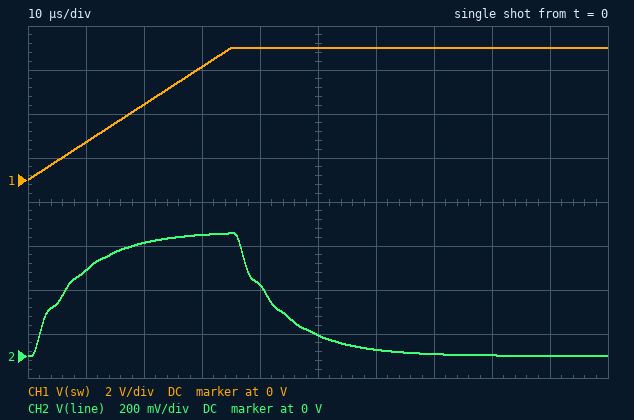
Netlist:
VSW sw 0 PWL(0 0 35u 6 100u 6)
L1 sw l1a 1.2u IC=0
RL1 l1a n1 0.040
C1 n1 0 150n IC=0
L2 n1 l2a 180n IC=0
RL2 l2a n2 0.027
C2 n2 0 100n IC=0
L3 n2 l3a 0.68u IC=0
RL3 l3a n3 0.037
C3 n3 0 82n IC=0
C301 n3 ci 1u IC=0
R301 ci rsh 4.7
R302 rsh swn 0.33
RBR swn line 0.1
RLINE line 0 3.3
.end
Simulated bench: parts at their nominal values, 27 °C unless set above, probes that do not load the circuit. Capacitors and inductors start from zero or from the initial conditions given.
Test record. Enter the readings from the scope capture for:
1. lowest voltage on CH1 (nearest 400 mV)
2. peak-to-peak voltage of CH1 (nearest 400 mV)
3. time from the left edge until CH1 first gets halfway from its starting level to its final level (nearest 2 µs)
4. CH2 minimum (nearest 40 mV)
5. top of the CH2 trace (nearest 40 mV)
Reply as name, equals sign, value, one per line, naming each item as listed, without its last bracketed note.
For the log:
lowest voltage on CH1 = 0 V
peak-to-peak voltage of CH1 = 6.0 V
time from the left edge until CH1 first gets halfway from its starting level to its final level = 18 µs
CH2 minimum = 0 V
top of the CH2 trace = 560 mV
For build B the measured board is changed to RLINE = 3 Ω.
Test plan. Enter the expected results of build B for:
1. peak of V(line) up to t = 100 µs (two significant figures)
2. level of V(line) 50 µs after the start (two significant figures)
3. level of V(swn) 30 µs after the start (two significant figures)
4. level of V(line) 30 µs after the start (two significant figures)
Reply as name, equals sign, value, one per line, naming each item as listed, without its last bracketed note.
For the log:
peak of V(line) up to t = 100 µs = 510 mV
level of V(line) 50 µs after the start = 79 mV
level of V(swn) 30 µs after the start = 520 mV
level of V(line) 30 µs after the start = 500 mV
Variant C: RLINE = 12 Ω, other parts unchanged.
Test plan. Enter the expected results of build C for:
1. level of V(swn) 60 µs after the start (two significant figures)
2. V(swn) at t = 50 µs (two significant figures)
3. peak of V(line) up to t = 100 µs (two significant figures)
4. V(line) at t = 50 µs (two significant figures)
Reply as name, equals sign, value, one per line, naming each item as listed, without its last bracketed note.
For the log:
level of V(swn) 60 µs after the start = 420 mV
V(swn) at t = 50 µs = 750 mV
peak of V(line) up to t = 100 µs = 1.8 V
V(line) at t = 50 µs = 740 mV
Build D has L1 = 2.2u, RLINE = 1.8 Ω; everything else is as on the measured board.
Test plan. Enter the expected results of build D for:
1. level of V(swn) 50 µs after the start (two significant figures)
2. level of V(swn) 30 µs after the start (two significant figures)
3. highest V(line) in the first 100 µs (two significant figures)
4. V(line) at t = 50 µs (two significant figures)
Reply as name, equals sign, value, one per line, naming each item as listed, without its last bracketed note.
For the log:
level of V(swn) 50 µs after the start = 35 mV
level of V(swn) 30 µs after the start = 320 mV
highest V(line) in the first 100 µs = 310 mV
V(line) at t = 50 µs = 33 mV
